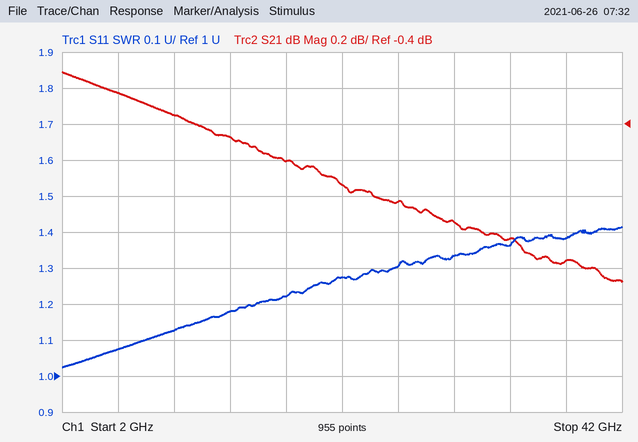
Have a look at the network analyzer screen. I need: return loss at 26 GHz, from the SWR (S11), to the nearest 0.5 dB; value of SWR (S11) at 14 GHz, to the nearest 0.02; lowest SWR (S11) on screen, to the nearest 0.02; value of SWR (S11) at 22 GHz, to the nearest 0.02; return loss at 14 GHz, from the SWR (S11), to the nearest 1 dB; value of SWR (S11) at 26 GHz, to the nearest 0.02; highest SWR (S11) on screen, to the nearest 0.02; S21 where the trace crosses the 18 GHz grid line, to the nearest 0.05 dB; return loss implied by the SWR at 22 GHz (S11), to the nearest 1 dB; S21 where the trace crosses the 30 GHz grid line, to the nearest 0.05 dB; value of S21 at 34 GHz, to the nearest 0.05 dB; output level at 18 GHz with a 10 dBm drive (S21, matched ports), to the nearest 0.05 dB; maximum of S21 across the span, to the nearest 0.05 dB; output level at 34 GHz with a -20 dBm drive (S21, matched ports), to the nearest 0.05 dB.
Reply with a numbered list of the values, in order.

1. 17.5 dB
2. 1.18
3. 1.02
4. 1.28
5. 22 dB
6. 1.30
7. 1.42
8. -0.60 dB
9. 18 dB
10. -0.95 dB
11. -1.05 dB
12. 9.40 dBm
13. -0.10 dB
14. -21.05 dBm
